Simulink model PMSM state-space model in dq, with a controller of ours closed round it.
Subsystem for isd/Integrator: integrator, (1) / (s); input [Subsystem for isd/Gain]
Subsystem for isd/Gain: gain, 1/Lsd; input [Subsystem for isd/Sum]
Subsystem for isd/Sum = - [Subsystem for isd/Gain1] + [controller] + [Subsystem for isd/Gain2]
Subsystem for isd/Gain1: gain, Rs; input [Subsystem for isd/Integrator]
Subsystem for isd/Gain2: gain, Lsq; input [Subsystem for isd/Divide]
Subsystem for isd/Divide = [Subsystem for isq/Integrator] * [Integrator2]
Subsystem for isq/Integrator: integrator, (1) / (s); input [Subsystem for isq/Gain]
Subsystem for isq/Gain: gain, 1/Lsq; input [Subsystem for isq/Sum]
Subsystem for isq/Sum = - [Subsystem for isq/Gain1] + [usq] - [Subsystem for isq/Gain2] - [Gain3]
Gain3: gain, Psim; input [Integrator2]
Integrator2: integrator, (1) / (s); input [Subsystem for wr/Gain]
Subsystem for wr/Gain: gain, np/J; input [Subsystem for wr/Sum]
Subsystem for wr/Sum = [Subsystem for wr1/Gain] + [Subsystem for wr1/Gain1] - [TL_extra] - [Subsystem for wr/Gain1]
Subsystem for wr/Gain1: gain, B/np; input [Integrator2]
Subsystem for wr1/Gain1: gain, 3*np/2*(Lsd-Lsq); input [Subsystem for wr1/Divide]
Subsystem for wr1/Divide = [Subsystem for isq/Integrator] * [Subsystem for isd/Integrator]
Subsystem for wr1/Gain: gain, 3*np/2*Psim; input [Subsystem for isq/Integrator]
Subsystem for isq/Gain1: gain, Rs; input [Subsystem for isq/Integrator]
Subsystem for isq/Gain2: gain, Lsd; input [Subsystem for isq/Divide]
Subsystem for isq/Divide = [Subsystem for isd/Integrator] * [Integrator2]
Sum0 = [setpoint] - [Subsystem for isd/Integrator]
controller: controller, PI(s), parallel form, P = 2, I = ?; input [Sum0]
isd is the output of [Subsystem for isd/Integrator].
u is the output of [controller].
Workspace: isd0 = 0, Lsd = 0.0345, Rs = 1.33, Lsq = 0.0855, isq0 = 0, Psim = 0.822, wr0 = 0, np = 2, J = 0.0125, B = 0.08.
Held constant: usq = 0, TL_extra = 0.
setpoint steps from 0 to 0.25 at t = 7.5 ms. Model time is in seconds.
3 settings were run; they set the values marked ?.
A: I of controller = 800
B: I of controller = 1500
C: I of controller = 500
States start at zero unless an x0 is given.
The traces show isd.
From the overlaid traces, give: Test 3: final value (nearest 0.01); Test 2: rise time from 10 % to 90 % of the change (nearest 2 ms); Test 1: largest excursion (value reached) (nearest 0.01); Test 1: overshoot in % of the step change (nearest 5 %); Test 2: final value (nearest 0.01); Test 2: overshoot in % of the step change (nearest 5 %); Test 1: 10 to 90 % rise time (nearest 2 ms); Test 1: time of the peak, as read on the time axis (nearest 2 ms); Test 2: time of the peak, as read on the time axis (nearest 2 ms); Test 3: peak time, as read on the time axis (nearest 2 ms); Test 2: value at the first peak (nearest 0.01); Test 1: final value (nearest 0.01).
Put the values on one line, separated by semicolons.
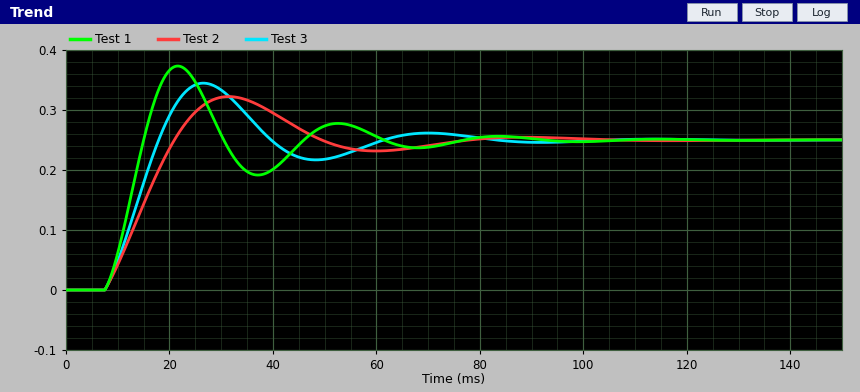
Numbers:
0.25; 10 ms; 0.37; 50 %; 0.25; 30 %; 6 ms; 22 ms; 32 ms; 26 ms; 0.32; 0.25
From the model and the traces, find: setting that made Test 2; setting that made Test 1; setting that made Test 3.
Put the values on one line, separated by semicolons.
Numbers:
C; B; A
